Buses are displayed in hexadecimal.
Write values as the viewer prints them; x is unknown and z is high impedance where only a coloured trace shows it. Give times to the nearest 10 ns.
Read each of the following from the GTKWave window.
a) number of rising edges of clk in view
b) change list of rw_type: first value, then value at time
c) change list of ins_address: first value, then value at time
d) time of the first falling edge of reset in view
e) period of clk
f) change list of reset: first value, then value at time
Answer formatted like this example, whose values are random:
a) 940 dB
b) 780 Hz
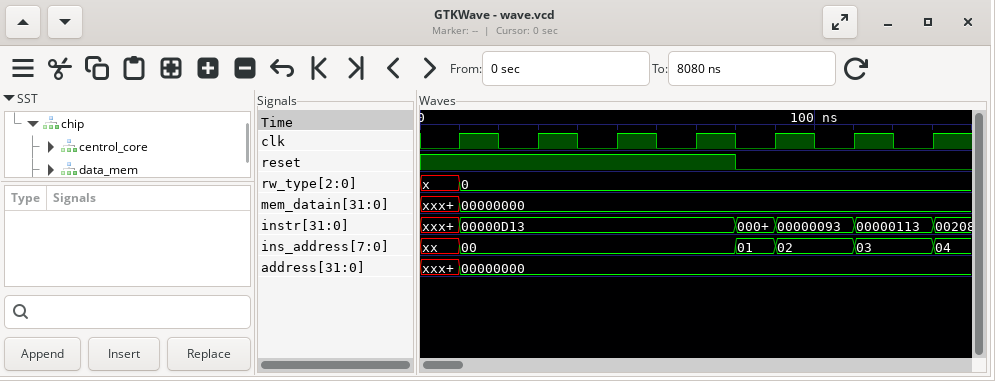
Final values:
a) 7
b) x, 0 at 10 ns
c) xx, 00 at 10 ns, 01 at 80 ns, 02 at 90 ns, 03 at 110 ns, 04 at 130 ns
d) 80 ns
e) 20 ns
f) 1, 0 at 80 ns
